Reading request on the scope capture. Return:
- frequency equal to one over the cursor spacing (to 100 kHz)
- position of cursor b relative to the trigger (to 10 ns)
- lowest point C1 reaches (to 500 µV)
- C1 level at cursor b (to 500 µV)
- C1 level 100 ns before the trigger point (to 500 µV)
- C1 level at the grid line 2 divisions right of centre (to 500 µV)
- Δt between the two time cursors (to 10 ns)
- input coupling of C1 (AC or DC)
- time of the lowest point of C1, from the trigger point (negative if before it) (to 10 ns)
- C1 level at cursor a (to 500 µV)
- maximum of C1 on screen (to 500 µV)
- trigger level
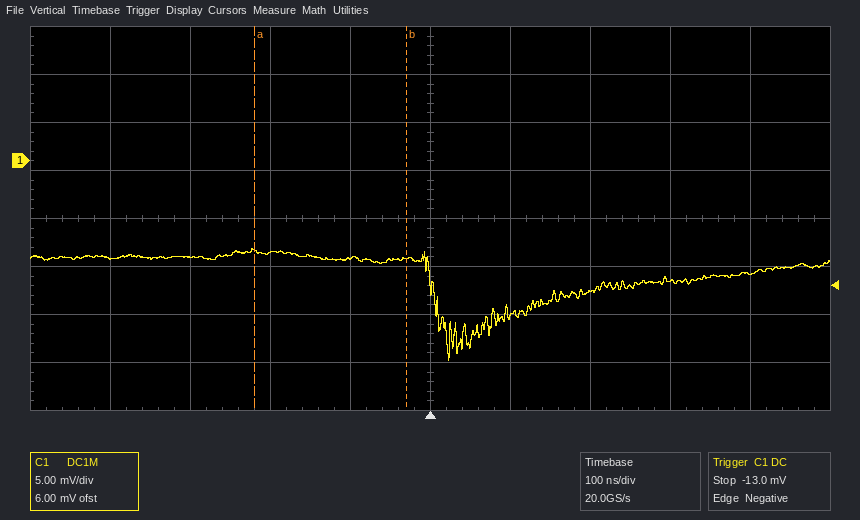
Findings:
5.3 MHz
-30 ns
-21.0 mV
-10.0 mV
-10.0 mV
-13.5 mV
190 ns
DC
+20 ns
-9.5 mV
-9.0 mV
-13.0 mV
